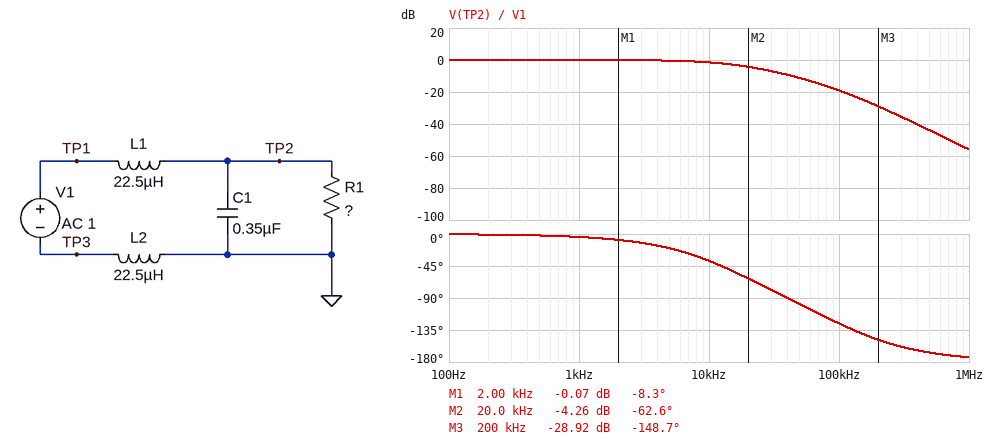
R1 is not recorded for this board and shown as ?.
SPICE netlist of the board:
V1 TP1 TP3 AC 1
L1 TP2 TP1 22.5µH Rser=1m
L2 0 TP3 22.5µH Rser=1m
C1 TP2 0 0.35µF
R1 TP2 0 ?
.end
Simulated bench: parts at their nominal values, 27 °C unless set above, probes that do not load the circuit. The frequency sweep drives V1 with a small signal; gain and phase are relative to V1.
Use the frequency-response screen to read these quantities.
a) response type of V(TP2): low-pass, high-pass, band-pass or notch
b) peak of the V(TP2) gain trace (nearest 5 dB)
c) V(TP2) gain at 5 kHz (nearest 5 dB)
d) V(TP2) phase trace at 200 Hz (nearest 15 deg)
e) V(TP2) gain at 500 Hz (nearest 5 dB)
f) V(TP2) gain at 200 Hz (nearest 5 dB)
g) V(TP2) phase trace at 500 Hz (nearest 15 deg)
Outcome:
low-pass
0 dB
0 dB
0 deg
0 dB
0 dB
0 deg
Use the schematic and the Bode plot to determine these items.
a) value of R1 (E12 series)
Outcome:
3.9 Ω
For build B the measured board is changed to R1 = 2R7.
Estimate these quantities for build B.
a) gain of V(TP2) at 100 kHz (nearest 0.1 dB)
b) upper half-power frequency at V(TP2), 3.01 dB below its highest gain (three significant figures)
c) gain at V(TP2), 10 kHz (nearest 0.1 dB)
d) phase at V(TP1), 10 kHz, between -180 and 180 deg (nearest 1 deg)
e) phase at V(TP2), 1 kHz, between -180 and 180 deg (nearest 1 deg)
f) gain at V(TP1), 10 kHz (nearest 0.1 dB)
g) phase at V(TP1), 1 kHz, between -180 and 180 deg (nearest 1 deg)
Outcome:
-21.4 dB
10.1 kHz
-3.0 dB
-20 deg
-6 deg
-2.1 dB
-3 deg
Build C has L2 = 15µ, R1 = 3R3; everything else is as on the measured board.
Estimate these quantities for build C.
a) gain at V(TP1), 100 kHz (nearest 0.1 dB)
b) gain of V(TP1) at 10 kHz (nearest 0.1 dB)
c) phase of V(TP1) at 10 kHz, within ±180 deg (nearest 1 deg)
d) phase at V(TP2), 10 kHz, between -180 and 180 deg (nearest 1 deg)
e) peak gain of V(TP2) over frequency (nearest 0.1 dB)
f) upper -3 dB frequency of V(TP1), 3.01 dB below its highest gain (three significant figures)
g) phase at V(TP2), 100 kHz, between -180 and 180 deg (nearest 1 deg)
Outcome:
-4.8 dB
-1.0 dB
-13 deg
-37 deg
0 dB
24.4 kHz
-120 deg
